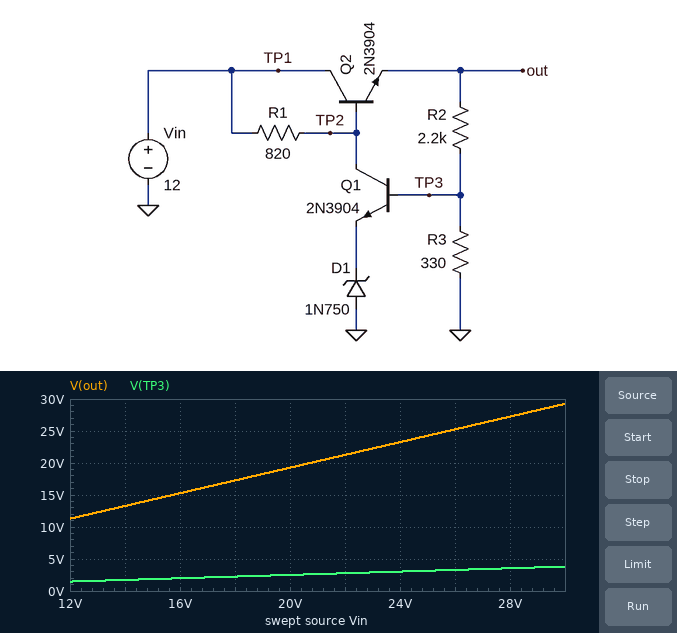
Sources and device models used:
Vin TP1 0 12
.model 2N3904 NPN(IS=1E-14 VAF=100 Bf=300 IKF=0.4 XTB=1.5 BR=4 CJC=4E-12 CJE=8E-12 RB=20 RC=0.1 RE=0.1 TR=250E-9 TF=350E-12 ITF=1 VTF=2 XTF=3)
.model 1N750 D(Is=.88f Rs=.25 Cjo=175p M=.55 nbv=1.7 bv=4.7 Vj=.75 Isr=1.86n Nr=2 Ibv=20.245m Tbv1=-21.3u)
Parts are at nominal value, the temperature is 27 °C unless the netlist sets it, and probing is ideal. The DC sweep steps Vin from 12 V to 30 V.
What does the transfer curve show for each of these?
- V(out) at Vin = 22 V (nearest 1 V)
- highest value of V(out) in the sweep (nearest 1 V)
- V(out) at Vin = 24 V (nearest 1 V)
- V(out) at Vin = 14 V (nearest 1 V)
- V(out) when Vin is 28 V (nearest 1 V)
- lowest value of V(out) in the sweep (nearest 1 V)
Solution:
21 V
29 V
23 V
13 V
27 V
11 V
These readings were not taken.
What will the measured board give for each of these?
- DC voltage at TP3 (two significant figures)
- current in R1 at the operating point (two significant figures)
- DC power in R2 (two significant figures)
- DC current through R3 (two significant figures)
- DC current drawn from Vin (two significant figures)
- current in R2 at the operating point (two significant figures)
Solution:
1.5 V
15 µA
44 mW
4.5 mA
4.5 mA
4.5 mA
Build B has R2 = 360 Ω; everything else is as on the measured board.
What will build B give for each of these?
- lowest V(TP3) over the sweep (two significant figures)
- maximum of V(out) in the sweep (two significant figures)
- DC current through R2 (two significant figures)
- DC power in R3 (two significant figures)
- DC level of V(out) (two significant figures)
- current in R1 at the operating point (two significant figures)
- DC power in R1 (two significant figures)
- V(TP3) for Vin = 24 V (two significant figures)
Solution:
5.2 V
11 V
16 mA
81 mW
11 V
550 µA
250 µW
5.4 V
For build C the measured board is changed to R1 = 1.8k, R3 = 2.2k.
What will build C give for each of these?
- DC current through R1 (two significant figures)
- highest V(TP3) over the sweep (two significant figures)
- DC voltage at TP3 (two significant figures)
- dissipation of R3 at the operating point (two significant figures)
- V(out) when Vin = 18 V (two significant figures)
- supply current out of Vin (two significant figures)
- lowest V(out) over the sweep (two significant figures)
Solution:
540 µA
5.4 V
5.2 V
12 mW
11 V
2.9 mA
10 V
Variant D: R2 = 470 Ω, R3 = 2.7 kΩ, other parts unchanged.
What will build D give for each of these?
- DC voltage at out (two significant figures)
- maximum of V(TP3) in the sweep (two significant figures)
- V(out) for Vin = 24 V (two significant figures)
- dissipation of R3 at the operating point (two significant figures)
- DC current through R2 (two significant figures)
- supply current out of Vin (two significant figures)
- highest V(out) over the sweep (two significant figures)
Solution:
6.3 V
5.5 V
6.4 V
11 mW
2.0 mA
8.1 mA
6.5 V
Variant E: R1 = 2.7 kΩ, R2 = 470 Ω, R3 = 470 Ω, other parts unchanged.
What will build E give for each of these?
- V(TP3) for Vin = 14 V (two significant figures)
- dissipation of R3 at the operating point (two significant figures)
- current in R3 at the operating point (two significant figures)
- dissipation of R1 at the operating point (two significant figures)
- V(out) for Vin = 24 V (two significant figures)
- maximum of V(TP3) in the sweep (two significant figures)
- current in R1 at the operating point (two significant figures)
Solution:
5.2 V
56 mW
11 mA
360 µW
11 V
5.4 V
370 µA
